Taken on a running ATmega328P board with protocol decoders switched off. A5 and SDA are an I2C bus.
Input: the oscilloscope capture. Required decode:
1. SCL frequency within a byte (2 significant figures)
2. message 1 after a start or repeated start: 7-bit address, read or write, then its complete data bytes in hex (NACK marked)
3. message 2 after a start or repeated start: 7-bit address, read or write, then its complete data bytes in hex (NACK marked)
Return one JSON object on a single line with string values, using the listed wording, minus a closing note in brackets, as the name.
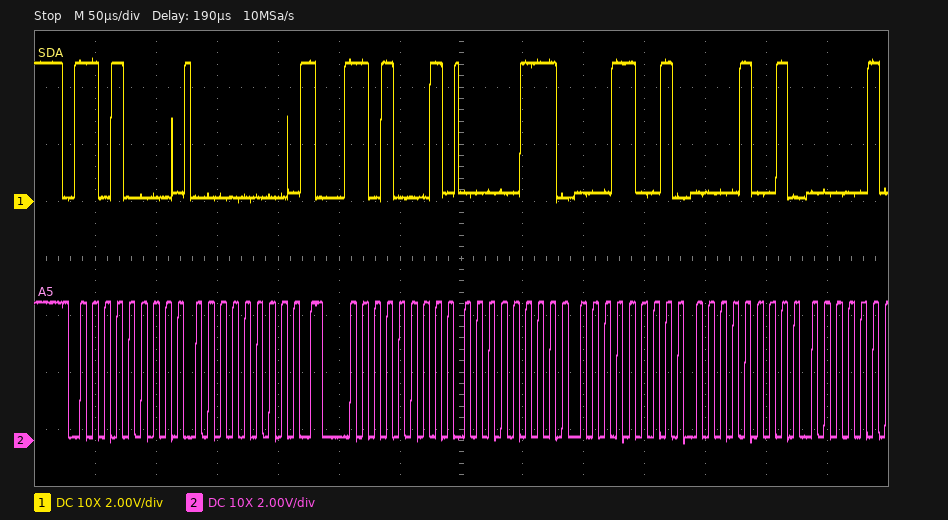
{"SCL frequency within a byte": "100 kHz", "message 1 after a start or repeated start: 7-bit address, read or write, then its complete data bytes in hex": "0x68 write: 00", "message 2 after a start or repeated start: 7-bit address, read or write, then its complete data bytes in hex": "0x68 read: 07 19 09"}
